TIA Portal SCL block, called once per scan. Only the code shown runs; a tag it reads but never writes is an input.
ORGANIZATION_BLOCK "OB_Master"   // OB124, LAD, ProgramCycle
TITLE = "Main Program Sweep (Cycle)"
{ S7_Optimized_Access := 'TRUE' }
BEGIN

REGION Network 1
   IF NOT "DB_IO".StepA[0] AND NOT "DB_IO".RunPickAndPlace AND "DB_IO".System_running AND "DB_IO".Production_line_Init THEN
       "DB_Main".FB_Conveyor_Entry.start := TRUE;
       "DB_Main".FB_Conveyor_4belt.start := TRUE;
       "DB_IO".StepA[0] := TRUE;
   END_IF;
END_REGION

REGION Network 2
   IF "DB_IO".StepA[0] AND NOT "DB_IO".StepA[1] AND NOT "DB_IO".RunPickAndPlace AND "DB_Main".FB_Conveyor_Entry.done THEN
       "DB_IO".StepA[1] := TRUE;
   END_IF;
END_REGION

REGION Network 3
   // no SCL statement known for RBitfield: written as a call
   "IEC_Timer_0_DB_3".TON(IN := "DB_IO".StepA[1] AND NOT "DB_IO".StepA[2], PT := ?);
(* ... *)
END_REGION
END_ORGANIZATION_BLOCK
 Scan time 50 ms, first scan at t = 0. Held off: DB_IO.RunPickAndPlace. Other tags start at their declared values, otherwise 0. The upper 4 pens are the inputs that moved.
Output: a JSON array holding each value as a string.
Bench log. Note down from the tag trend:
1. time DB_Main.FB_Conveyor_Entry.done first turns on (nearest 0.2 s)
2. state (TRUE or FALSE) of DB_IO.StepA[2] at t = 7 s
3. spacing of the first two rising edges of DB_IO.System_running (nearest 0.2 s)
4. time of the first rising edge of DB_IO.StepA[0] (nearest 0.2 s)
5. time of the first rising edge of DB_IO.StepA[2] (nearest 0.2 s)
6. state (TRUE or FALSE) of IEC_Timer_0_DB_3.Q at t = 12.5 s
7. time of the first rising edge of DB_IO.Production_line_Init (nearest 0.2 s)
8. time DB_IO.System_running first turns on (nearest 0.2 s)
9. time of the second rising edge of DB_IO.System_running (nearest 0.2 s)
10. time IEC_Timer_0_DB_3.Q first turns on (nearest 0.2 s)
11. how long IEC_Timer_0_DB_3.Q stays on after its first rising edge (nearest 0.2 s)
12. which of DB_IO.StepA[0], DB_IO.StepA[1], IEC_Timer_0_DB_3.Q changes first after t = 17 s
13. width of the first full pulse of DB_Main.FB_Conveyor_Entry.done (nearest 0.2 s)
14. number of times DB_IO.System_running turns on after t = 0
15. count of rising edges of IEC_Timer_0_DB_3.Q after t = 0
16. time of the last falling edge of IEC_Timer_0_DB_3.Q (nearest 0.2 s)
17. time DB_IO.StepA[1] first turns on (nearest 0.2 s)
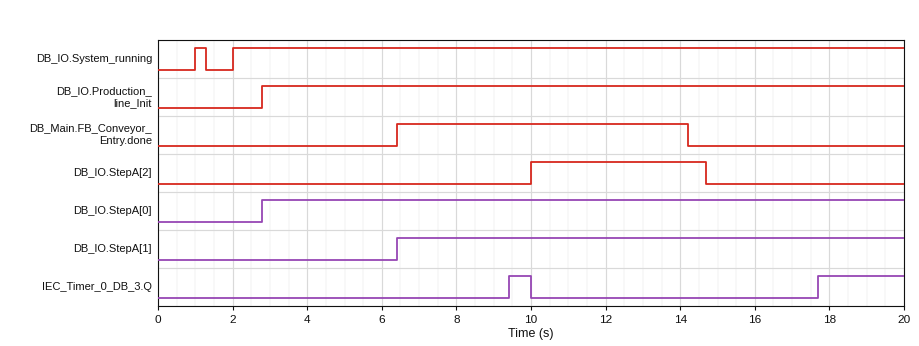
["6.4 s", "FALSE", "1.0 s", "2.8 s", "10.0 s", "FALSE", "2.8 s", "1.0 s", "2.0 s", "9.4 s", "0.6 s", "IEC_Timer_0_DB_3.Q", "7.8 s", "2", "2", "10.0 s", "6.4 s"]
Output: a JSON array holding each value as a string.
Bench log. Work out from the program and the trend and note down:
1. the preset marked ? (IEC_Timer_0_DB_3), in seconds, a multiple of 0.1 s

["3.0 s"]
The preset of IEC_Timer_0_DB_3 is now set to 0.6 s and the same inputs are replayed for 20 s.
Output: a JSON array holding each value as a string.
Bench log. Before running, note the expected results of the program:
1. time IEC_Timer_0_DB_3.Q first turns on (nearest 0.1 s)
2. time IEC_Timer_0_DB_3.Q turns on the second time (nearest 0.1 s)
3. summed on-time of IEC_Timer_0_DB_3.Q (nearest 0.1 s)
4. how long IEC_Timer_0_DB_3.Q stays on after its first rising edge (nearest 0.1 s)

["7.0 s", "15.3 s", "7.7 s", "3.0 s"]
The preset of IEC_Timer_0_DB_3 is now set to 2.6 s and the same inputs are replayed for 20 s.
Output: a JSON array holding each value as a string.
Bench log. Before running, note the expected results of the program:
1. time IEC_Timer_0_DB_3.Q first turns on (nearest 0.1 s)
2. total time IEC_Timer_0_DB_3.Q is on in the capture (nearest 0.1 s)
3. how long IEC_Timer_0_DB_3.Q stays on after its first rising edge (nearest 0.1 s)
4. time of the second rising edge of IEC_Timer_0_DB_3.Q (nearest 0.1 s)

["9.0 s", "3.7 s", "1.0 s", "17.3 s"]
